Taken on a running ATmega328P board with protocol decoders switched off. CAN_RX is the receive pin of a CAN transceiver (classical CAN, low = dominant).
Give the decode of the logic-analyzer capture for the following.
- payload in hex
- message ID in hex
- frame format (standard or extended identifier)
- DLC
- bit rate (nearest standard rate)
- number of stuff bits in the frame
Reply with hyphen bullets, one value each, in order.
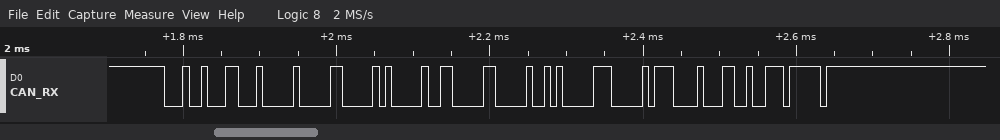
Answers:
- 01 02 03 04 05 06 07 08
- 0x123
- standard
- 8
- 125 kbit/s
- 8
